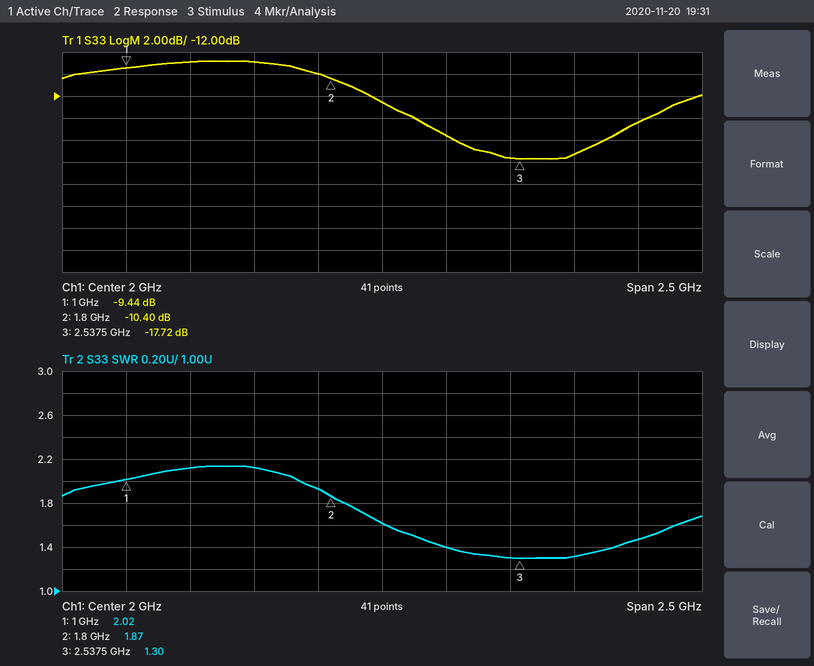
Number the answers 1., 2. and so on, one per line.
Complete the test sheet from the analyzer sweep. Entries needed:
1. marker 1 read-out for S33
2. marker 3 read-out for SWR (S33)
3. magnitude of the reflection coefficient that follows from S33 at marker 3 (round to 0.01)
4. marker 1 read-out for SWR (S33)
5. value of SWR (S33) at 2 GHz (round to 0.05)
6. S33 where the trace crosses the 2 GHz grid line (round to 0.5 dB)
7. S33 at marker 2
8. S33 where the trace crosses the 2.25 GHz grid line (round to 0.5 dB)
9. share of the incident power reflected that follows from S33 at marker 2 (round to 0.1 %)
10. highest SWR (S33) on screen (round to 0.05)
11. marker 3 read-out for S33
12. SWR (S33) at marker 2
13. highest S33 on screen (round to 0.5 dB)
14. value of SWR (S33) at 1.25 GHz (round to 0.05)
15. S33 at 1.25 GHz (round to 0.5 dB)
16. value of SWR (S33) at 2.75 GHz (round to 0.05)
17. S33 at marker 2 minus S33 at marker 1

1. -9.44 dB
2. 1.30
3. 0.13
4. 2.02
5. 1.60
6. -12.5 dB
7. -10.40 dB
8. -15.5 dB
9. 9.1 %
10. 2.15
11. -17.72 dB
12. 1.87
13. -9.0 dB
14. 2.10
15. -9.0 dB
16. 1.30
17. -0.96 dB
